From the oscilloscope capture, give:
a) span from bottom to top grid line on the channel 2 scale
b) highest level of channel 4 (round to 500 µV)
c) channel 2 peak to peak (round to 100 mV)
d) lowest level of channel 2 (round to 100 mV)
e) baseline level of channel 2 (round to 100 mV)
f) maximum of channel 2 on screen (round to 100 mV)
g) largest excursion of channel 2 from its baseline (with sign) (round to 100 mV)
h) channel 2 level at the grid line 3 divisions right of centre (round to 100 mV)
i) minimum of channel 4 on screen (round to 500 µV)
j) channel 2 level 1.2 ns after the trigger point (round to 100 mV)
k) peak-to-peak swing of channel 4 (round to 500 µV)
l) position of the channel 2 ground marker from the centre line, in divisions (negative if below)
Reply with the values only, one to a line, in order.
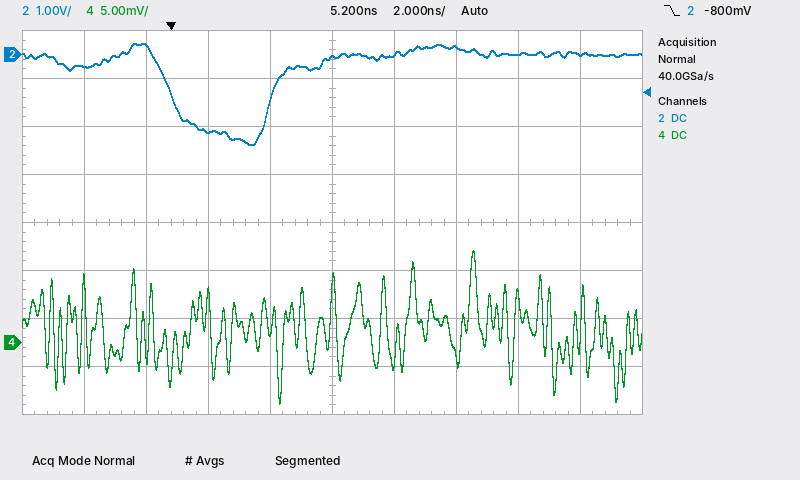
8 V
9.5 mV
2.1 V
-1.9 V
0.0 V
200 mV
-1.9 V
0.0 V
-6.5 mV
-1.6 V
16.0 mV
+3.5 div
